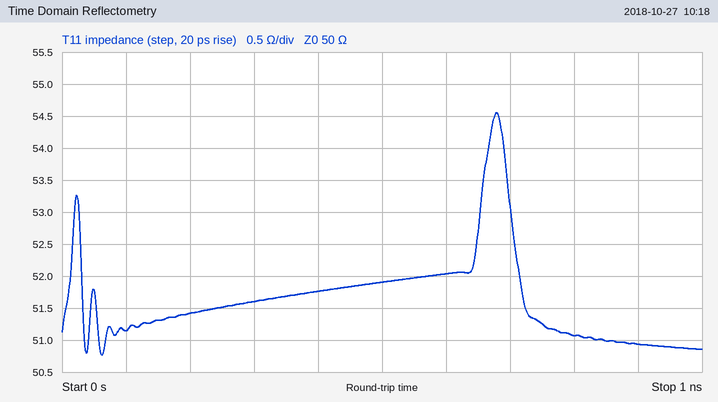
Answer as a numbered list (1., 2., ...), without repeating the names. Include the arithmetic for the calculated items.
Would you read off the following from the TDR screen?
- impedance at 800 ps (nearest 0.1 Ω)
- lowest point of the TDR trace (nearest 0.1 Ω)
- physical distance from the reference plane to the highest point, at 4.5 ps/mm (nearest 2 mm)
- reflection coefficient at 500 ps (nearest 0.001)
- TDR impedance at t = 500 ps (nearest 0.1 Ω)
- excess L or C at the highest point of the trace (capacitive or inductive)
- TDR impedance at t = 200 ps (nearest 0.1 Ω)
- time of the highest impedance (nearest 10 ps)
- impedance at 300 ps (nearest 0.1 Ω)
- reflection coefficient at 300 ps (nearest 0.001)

1. 51.1 Ω
2. 50.8 Ω
3. 680 ps / 2 / 4.5 ps/mm ≈ 76 mm
4. (51.9 − 50)/(51.9 + 50) ≈ +0.019
5. 51.9 Ω
6. inductive
7. 51.4 Ω
8. 680 ps
9. 51.6 Ω
10. (51.6 − 50)/(51.6 + 50) ≈ +0.016
